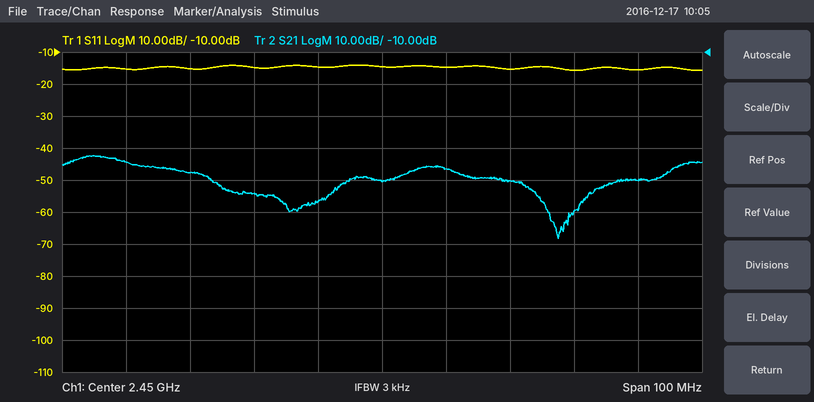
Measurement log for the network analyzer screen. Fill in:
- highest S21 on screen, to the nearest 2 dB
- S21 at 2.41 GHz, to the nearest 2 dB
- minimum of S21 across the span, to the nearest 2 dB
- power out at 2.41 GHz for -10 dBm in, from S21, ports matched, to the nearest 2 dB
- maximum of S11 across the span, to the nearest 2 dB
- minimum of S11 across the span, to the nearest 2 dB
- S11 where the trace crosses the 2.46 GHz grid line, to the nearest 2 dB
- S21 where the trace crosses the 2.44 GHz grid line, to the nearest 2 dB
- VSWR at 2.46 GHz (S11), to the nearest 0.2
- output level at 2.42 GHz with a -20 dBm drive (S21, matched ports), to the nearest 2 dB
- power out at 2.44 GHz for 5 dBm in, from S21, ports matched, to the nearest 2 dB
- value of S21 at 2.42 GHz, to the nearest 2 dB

-42 dB
-44 dB
-68 dB
-54 dBm
-14 dB
-16 dB
-14 dB
-56 dB
1.4
-68 dBm
-52 dBm
-48 dB
